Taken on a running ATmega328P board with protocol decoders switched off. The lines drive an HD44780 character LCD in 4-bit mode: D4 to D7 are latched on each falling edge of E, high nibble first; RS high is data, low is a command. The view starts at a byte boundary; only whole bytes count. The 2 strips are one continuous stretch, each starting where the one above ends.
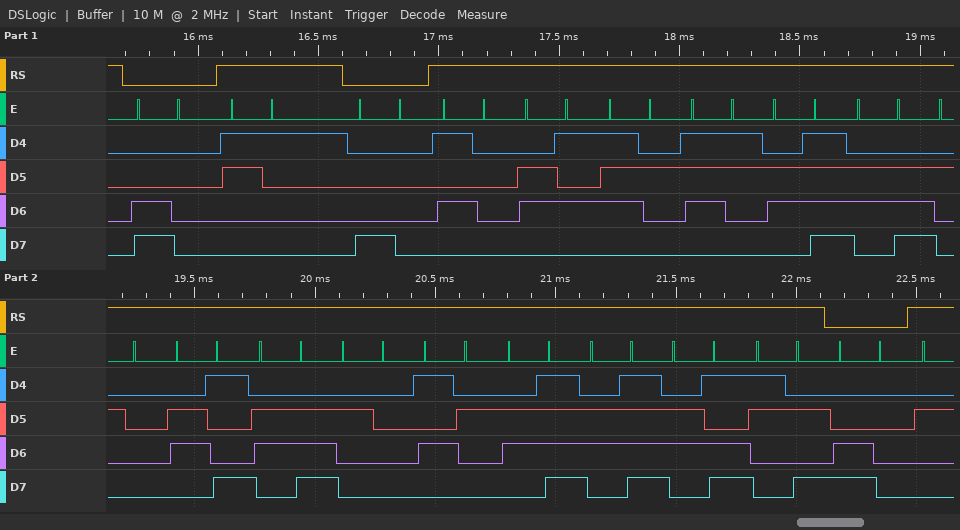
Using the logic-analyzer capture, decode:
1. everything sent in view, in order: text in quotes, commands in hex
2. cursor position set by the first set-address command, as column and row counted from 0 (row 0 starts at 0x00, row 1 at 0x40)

0xC0 "1" 0x80 "Person in Room:" 0xC0
column 0, row 1
